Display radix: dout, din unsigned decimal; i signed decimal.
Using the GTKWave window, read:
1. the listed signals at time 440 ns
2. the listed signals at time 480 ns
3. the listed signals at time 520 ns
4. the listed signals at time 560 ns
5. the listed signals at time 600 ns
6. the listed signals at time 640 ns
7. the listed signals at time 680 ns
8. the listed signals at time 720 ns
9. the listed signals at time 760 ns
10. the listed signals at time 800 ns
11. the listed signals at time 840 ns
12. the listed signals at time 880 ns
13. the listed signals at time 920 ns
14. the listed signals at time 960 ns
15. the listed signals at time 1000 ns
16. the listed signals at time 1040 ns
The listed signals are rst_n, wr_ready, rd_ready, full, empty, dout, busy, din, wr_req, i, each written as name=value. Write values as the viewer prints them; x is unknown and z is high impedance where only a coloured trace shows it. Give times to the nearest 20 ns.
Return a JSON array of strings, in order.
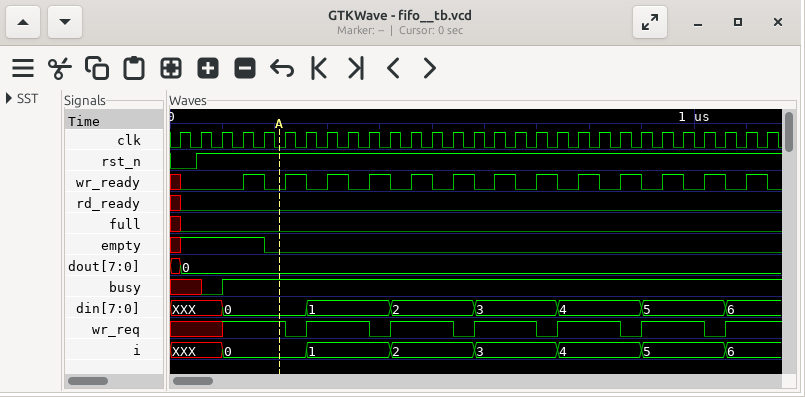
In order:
["rst_n=1, wr_ready=0, rd_ready=0, full=0, empty=0, dout=0, busy=1, din=2, wr_req=1, i=2", "rst_n=1, wr_ready=1, rd_ready=0, full=0, empty=0, dout=0, busy=1, din=2, wr_req=1, i=2", "rst_n=1, wr_ready=0, rd_ready=0, full=0, empty=0, dout=0, busy=1, din=2, wr_req=1, i=2", "rst_n=1, wr_ready=1, rd_ready=0, full=0, empty=0, dout=0, busy=1, din=2, wr_req=0, i=2", "rst_n=1, wr_ready=0, rd_ready=0, full=0, empty=0, dout=0, busy=1, din=3, wr_req=1, i=3", "rst_n=1, wr_ready=1, rd_ready=0, full=0, empty=0, dout=0, busy=1, din=3, wr_req=1, i=3", "rst_n=1, wr_ready=0, rd_ready=0, full=0, empty=0, dout=0, busy=1, din=3, wr_req=1, i=3", "rst_n=1, wr_ready=1, rd_ready=0, full=0, empty=0, dout=0, busy=1, din=3, wr_req=0, i=3", "rst_n=1, wr_ready=0, rd_ready=0, full=0, empty=0, dout=0, busy=1, din=4, wr_req=1, i=4", "rst_n=1, wr_ready=1, rd_ready=0, full=0, empty=0, dout=0, busy=1, din=4, wr_req=1, i=4", "rst_n=1, wr_ready=0, rd_ready=0, full=0, empty=0, dout=0, busy=1, din=4, wr_req=1, i=4", "rst_n=1, wr_ready=1, rd_ready=0, full=0, empty=0, dout=0, busy=1, din=4, wr_req=0, i=4", "rst_n=1, wr_ready=0, rd_ready=0, full=0, empty=0, dout=0, busy=1, din=5, wr_req=1, i=5", "rst_n=1, wr_ready=1, rd_ready=0, full=0, empty=0, dout=0, busy=1, din=5, wr_req=1, i=5", "rst_n=1, wr_ready=0, rd_ready=0, full=0, empty=0, dout=0, busy=1, din=5, wr_req=1, i=5", "rst_n=1, wr_ready=1, rd_ready=0, full=0, empty=0, dout=0, busy=1, din=5, wr_req=0, i=5"]
